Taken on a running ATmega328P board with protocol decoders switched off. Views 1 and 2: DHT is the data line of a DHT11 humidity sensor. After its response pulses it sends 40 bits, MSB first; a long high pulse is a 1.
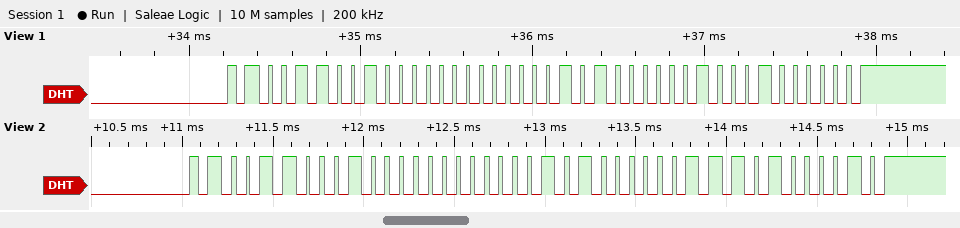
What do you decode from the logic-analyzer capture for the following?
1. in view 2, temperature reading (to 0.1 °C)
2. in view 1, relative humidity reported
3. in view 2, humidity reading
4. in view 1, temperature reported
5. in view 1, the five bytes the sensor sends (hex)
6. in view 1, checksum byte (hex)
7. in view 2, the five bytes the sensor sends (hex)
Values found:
10.7 °C
50 %
49 %
10.4 °C
32 00 0A 04 40
0x40
31 00 0A 07 42
